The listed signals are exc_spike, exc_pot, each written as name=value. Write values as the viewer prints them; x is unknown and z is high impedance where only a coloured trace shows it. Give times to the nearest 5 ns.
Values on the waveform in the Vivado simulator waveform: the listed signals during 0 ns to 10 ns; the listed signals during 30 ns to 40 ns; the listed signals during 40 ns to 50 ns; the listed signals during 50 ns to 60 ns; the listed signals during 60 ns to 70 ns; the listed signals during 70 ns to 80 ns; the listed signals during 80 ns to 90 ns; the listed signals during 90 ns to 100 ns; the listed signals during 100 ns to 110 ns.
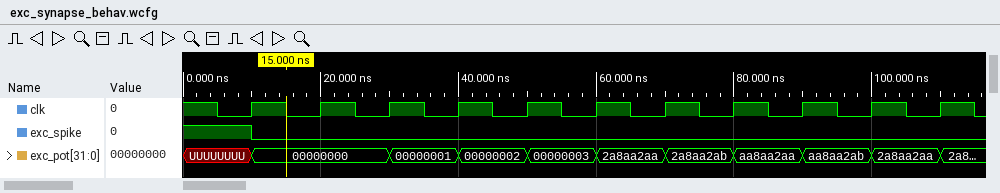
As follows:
exc_spike=1, exc_pot=UUUUUUUU
exc_spike=0, exc_pot=00000001
exc_spike=0, exc_pot=00000002
exc_spike=0, exc_pot=00000003
exc_spike=0, exc_pot=2a8aa2aa
exc_spike=0, exc_pot=2a8aa2ab
exc_spike=0, exc_pot=aa8aa2aa
exc_spike=0, exc_pot=aa8aa2ab
exc_spike=0, exc_pot=2a8aa2aa
